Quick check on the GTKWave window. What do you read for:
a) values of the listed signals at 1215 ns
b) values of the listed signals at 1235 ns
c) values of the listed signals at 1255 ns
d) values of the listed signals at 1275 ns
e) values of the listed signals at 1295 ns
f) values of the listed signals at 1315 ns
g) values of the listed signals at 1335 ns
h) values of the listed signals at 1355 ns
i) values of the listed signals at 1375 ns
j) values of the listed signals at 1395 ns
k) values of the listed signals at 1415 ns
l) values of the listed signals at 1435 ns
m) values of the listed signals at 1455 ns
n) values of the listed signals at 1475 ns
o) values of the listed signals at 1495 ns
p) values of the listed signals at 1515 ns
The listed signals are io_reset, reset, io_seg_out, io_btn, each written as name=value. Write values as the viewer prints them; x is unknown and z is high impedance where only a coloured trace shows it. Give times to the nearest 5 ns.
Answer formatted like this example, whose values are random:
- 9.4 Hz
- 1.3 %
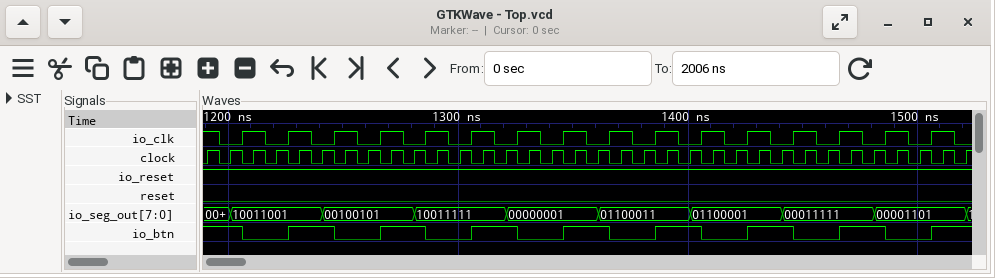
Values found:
- io_reset=1, reset=0, io_seg_out=10011001, io_btn=0
- io_reset=1, reset=0, io_seg_out=10011001, io_btn=1
- io_reset=1, reset=0, io_seg_out=00100101, io_btn=0
- io_reset=1, reset=0, io_seg_out=00100101, io_btn=1
- io_reset=1, reset=0, io_seg_out=10011111, io_btn=0
- io_reset=1, reset=0, io_seg_out=10011111, io_btn=1
- io_reset=1, reset=0, io_seg_out=00000001, io_btn=0
- io_reset=1, reset=0, io_seg_out=00000001, io_btn=1
- io_reset=1, reset=0, io_seg_out=01100011, io_btn=0
- io_reset=1, reset=0, io_seg_out=01100011, io_btn=1
- io_reset=1, reset=0, io_seg_out=01100001, io_btn=0
- io_reset=1, reset=0, io_seg_out=01100001, io_btn=1
- io_reset=1, reset=0, io_seg_out=00011111, io_btn=0
- io_reset=1, reset=0, io_seg_out=00011111, io_btn=1
- io_reset=1, reset=0, io_seg_out=00001101, io_btn=0
- io_reset=1, reset=0, io_seg_out=00001101, io_btn=1
